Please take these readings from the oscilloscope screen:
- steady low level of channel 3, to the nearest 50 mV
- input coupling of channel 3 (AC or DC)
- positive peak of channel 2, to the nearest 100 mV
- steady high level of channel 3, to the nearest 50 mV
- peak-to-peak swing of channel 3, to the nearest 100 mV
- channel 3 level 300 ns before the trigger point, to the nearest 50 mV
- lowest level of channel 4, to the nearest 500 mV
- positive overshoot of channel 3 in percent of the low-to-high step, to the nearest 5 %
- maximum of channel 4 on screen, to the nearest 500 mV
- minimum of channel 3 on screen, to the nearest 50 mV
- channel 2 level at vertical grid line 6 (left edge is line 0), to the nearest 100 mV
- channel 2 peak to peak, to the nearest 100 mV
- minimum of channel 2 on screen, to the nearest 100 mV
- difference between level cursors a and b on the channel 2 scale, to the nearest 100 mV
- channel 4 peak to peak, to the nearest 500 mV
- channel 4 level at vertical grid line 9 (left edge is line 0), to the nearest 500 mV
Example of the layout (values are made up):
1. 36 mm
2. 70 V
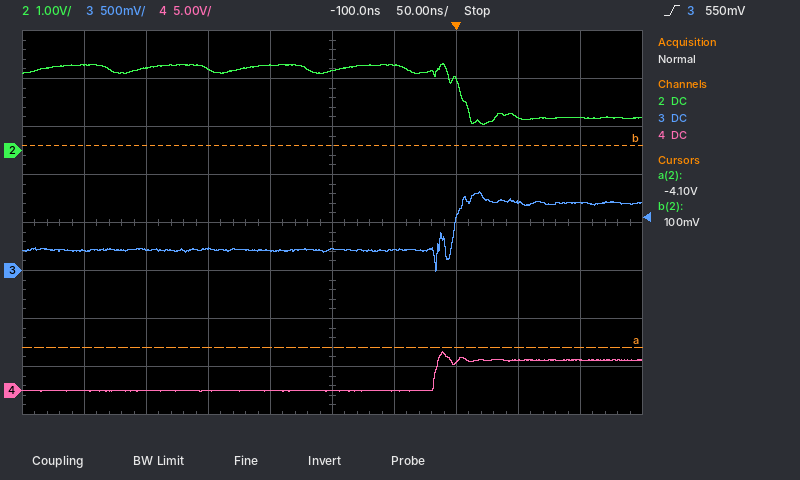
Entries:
1. 200 mV
2. DC
3. 1.8 V
4. 700 mV
5. 800 mV
6. 200 mV
7. 0.0 V
8. 25 %
9. 4.0 V
10. 0 mV
11. 1.8 V
12. 1.3 V
13. 500 mV
14. 4.2 V
15. 4.0 V
16. 3.0 V
